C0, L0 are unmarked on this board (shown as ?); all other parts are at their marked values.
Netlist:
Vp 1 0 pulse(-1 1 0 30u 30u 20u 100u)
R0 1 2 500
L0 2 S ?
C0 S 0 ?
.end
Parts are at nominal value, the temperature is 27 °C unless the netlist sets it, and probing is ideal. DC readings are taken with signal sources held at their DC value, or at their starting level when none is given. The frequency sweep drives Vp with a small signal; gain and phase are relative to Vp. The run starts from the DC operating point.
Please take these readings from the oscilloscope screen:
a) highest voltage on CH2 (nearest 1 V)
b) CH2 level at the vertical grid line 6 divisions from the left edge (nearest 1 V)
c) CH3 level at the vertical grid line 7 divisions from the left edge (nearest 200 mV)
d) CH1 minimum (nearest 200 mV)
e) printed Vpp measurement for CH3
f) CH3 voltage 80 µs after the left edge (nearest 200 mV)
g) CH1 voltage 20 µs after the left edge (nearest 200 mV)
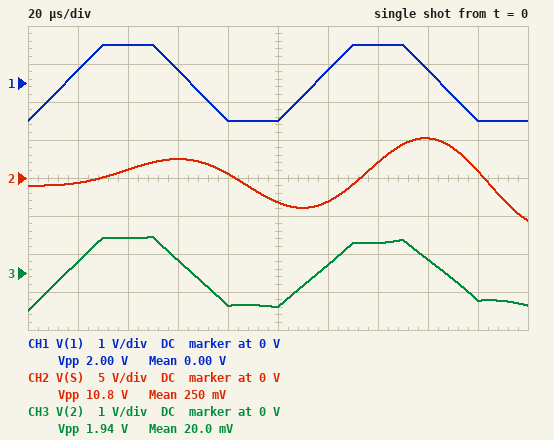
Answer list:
5 V
-3 V
800 mV
-1.0 V
1.94 V
-800 mV
400 mV
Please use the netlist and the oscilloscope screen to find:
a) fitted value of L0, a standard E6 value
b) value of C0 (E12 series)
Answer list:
150 mH
1.5 nF
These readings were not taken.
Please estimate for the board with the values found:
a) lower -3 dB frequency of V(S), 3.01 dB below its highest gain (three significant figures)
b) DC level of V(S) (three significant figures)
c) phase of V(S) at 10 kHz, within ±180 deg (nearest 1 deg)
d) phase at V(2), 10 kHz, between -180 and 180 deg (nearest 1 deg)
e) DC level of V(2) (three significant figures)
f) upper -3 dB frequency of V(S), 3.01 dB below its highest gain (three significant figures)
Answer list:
10.3 kHz
-1.00 V
-23 deg
-23 deg
-1.00 V
10.9 kHz
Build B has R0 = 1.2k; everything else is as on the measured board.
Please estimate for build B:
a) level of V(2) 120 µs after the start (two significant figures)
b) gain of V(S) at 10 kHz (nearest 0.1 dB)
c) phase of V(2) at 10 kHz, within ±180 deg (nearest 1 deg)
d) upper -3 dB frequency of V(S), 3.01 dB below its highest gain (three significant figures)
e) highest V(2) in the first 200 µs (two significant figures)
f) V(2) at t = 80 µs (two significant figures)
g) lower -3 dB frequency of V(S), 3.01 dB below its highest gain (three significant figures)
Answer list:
85 mV
16.0 dB
-45 deg
11.2 kHz
870 mV
-700 mV
9.91 kHz
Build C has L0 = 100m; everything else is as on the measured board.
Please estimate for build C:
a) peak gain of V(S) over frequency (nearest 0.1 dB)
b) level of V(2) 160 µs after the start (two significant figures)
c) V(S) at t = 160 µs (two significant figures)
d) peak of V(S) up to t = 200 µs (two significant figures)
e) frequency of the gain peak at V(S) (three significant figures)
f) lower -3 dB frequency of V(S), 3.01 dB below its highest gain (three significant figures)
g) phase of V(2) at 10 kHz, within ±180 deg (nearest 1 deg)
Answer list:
24.3 dB
510 mV
1.6 V
3.8 V
13.0 kHz
12.6 kHz
-7 deg
